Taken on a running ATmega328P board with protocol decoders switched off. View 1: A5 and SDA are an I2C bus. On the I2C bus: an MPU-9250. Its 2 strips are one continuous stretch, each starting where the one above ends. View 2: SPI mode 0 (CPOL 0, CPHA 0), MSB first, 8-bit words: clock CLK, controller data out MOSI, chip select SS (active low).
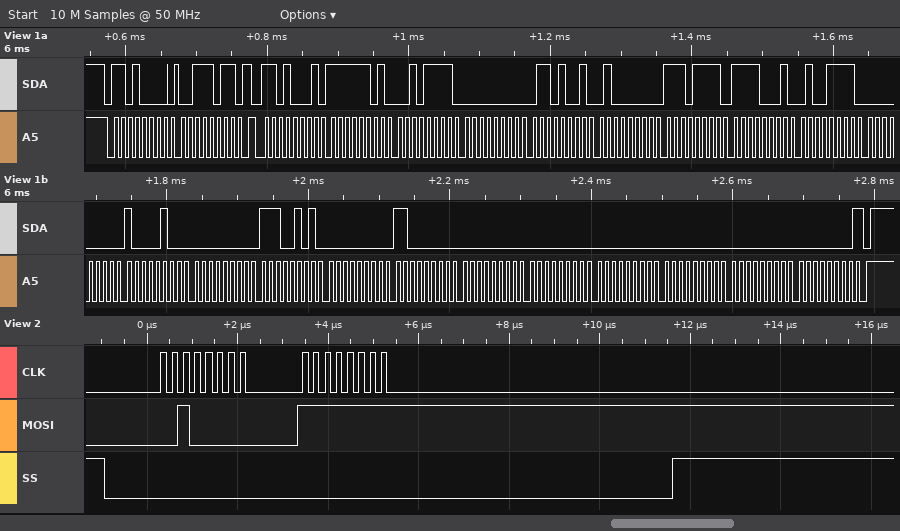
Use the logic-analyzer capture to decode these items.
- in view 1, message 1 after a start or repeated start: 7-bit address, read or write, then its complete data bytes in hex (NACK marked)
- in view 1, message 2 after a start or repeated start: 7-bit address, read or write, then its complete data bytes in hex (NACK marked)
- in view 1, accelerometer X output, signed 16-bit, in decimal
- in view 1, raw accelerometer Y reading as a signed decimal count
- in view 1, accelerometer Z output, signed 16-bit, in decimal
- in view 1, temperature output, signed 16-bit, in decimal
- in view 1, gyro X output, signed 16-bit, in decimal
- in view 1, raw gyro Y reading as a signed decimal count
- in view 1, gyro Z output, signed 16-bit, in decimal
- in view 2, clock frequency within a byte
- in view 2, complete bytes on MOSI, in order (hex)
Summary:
0x68 write: 3B
0x68 read: FD 2F 00 69 40 EF F1 4F 00 84 00 E5 00 C0 00 00 00 00 00 00 NACK
-721
105
16623
-3761
132
229
192
4 MHz
20 FF
